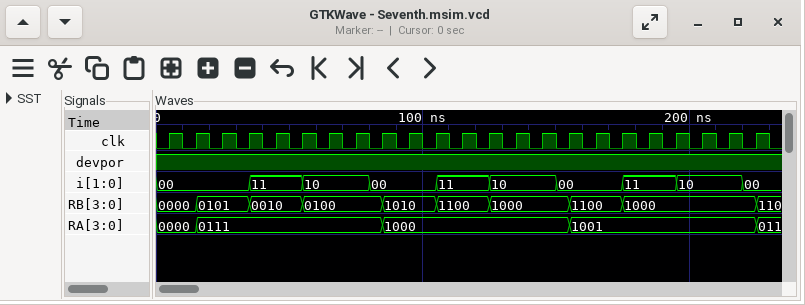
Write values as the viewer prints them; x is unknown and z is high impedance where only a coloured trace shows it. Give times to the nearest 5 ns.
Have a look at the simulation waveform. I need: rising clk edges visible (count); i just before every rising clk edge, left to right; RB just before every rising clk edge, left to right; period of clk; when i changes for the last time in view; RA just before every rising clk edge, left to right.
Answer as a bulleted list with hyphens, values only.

- 23
- 00, 00, 00, 00, 11, 11, 10, 10, 00, 00, 00, 11, 11, 10, 10, 00, 00, 00, 11, 11, 10, 10, 00
- 0000, 0000, 0101, 0101, 0010, 0010, 0100, 0100, 0100, 1010, 1010, 1100, 1100, 1000, 1000, 1000, 1100, 1100, 1000, 1000, 1000, 1000, 1000
- 10 ns
- 220 ns
- 0000, 0000, 0111, 0111, 0111, 0111, 0111, 0111, 0111, 1000, 1000, 1000, 1000, 1000, 1000, 1000, 1001, 1001, 1001, 1001, 1001, 1001, 1001
